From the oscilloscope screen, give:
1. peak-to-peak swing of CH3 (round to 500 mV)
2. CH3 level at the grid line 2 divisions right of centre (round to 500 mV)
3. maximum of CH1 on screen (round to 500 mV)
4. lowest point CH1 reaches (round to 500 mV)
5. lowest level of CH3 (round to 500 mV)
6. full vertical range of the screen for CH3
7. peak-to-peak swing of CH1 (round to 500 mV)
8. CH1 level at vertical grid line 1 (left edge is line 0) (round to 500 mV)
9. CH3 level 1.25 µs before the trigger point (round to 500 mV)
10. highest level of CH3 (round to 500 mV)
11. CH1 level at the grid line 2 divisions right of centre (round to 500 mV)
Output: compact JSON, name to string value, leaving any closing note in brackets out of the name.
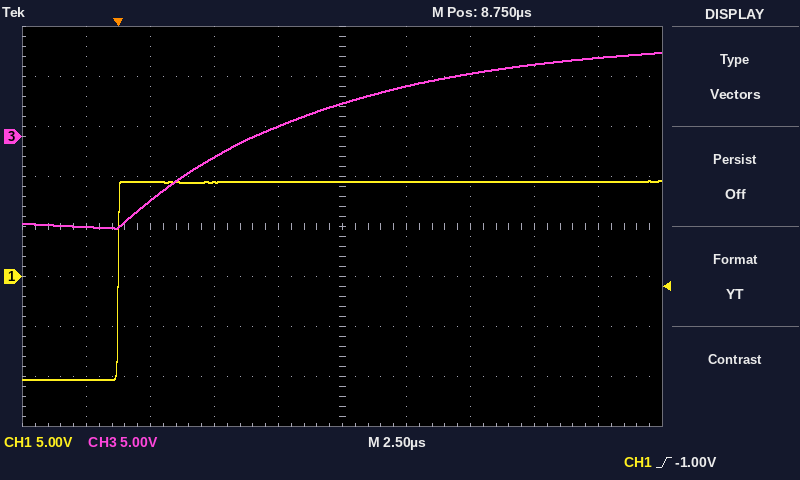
{"peak-to-peak swing of CH3": "17.5 V", "CH3 level at the grid line 2 divisions right of centre": "6.5 V", "maximum of CH1 on screen": "9.5 V", "lowest point CH1 reaches": "-10.5 V", "lowest level of CH3": "-9.0 V", "full vertical range of the screen for CH3": "40 V", "peak-to-peak swing of CH1": "20.0 V", "CH1 level at vertical grid line 1 (left edge is line 0)": "-10.5 V", "CH3 level 1.25 µs before the trigger point": "-9.0 V", "highest level of CH3": "8.5 V", "CH1 level at the grid line 2 divisions right of centre": "9.5 V"}
